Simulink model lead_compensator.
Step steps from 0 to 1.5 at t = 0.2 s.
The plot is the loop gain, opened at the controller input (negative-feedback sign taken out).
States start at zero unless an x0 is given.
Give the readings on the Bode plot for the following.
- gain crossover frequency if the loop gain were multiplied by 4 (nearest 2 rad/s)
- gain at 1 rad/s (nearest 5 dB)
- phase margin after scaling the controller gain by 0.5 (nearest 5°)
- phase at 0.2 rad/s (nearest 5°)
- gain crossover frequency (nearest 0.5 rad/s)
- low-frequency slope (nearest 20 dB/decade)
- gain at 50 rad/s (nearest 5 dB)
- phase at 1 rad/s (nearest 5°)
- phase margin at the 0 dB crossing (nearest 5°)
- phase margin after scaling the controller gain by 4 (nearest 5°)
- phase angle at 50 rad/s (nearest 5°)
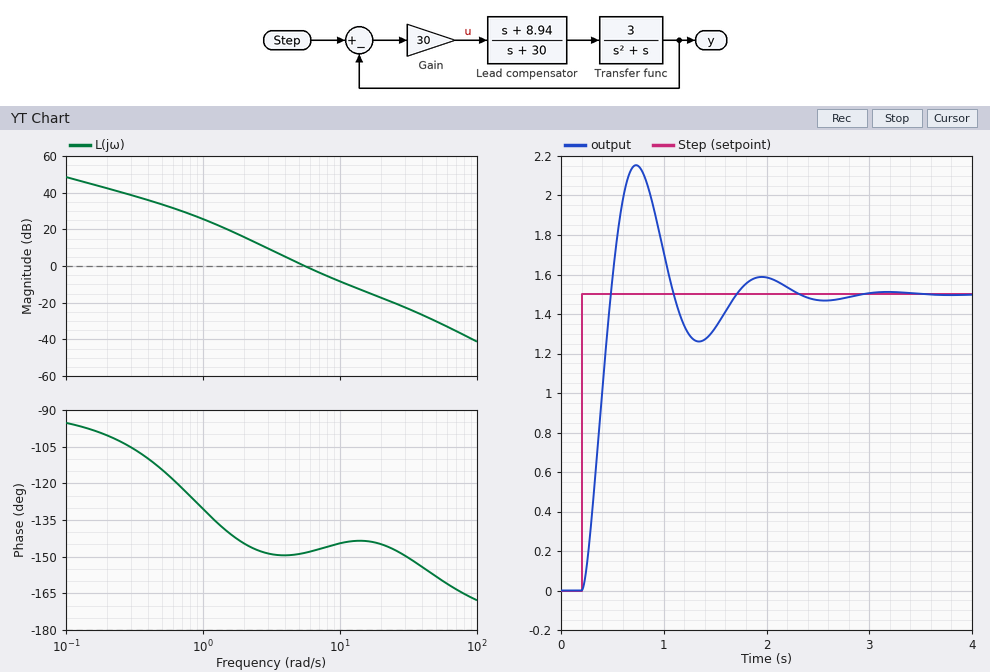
14 rad/s
25 dB
30°
-100°
5.5 rad/s
-20 dB/decade
-30 dB
-130°
30°
35°
-160°
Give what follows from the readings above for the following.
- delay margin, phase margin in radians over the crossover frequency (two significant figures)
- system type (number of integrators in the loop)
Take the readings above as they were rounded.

0.095 s
1
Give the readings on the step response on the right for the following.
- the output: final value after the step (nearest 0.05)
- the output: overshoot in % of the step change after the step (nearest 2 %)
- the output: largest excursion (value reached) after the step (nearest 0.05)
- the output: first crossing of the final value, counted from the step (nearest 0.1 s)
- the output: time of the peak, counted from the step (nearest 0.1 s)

1.50
44 %
2.15
0.3 s
0.5 s
